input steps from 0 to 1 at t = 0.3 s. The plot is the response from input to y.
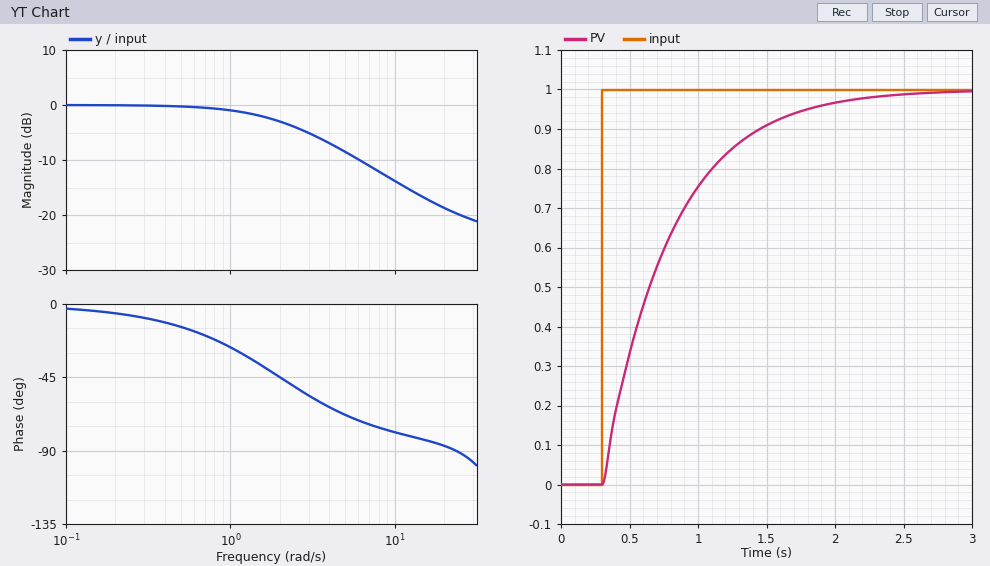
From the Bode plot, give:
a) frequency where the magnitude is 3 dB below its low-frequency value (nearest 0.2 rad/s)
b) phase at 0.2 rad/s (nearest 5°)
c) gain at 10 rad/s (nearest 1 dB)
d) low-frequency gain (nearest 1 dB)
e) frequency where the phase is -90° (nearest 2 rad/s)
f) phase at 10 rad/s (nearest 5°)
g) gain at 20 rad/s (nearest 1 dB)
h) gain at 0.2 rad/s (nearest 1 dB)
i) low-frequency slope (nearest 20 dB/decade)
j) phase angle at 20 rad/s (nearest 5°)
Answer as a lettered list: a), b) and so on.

a) 2.0 rad/s
b) -5°
c) -14 dB
d) 0 dB
e) 24 rad/s
f) -80°
g) -19 dB
h) 0 dB
i) 0 dB/decade
j) -85°
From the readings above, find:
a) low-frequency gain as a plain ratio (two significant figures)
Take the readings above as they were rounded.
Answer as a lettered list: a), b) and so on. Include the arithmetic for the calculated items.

a) 10^(0 / 20) = 1.0
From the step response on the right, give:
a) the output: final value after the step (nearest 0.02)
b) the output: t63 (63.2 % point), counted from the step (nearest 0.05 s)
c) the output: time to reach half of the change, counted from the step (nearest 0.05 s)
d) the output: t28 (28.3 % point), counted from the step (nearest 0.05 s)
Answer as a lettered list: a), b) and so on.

a) 1.00
b) 0.50 s
c) 0.35 s
d) 0.15 s
